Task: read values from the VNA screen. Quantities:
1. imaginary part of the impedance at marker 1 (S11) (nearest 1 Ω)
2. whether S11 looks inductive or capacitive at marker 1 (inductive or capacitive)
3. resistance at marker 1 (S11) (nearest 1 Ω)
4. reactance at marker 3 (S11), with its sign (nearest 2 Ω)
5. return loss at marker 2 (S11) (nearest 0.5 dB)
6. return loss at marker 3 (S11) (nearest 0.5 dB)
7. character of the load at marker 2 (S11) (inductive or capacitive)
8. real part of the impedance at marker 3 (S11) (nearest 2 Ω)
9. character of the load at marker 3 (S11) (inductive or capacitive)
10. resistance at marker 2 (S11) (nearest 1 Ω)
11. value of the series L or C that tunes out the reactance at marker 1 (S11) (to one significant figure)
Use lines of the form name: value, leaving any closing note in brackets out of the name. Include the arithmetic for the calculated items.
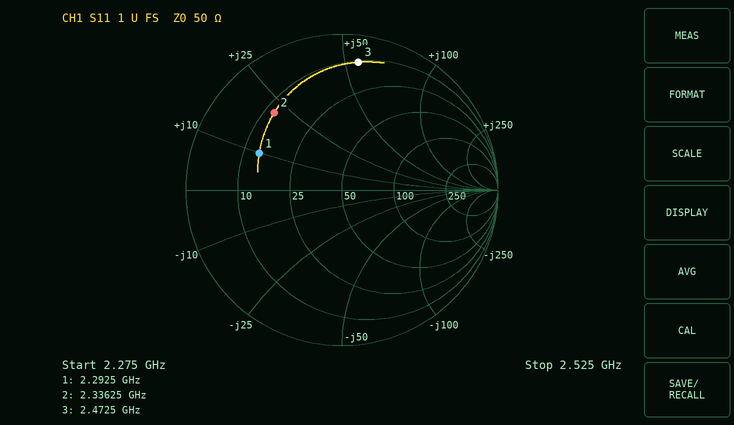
imaginary part of the impedance at marker 1 (S11): +10 Ω
whether S11 looks inductive or capacitive at marker 1: inductive
resistance at marker 1 (S11): 14 Ω
reactance at marker 3 (S11), with its sign: +56 Ω
return loss at marker 2 (S11): 3.5 dB
return loss at marker 3 (S11): 1.5 dB
character of the load at marker 2 (S11): inductive
real part of the impedance at marker 3 (S11): 10 Ω
character of the load at marker 3 (S11): inductive
resistance at marker 2 (S11): 12 Ω
value of the series L or C that tunes out the reactance at marker 1 (S11): C = 1/(2π × 2.2925 GHz × 10 Ω) ≈ 7 pF
